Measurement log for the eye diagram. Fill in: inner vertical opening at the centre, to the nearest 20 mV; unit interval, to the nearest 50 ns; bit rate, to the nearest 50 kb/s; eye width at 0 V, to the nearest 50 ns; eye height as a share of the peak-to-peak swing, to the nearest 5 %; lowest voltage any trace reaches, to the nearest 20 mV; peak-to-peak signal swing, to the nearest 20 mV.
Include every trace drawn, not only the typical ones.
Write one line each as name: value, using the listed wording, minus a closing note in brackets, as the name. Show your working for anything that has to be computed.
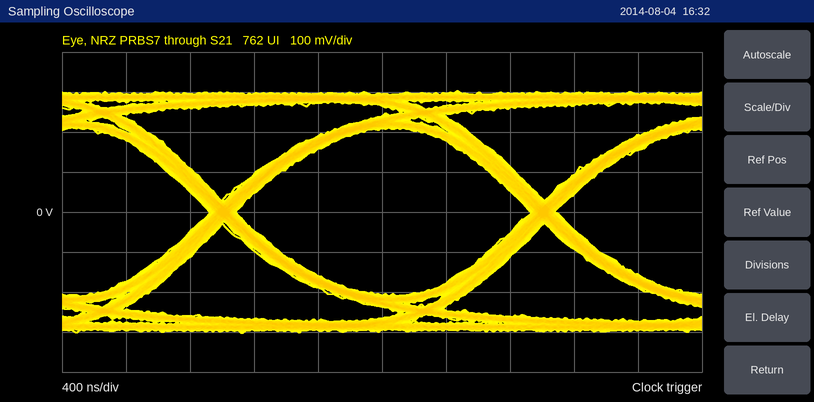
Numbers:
inner vertical opening at the centre, to the nearest 20 mV: 420 mV
unit interval, to the nearest 50 ns: 2.00 µs
bit rate, to the nearest 50 kb/s: 500 kb/s
eye width at 0 V, to the nearest 50 ns: 1.85 µs
eye height as a share of the peak-to-peak swing, to the nearest 5 %: 420 mV / 600 mV ≈ 70 %
lowest voltage any trace reaches, to the nearest 20 mV: -300 mV
peak-to-peak signal swing, to the nearest 20 mV: 600 mV
